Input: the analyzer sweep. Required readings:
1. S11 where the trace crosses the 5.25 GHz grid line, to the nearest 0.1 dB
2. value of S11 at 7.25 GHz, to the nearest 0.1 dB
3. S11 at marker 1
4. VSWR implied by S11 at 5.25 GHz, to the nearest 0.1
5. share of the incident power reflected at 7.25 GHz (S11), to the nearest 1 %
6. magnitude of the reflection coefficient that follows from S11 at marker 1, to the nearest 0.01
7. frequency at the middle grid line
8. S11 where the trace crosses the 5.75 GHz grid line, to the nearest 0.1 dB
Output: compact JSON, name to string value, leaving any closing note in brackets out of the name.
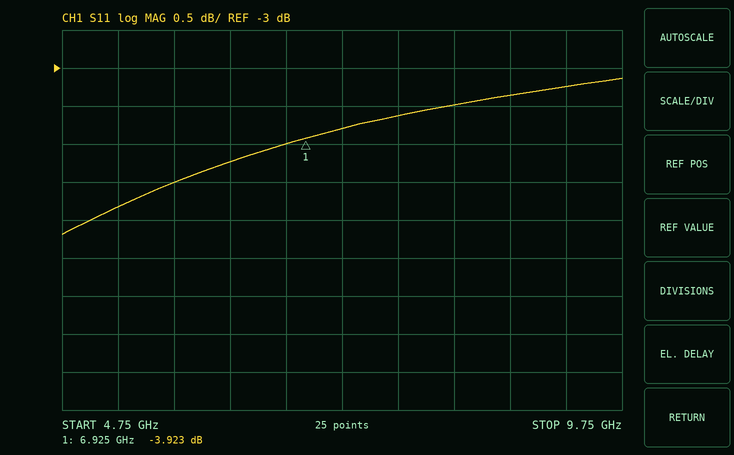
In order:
{"S11 where the trace crosses the 5.25 GHz grid line, to the nearest 0.1 dB": "-4.8 dB", "value of S11 at 7.25 GHz, to the nearest 0.1 dB": "-3.8 dB", "S11 at marker 1": "-3.923 dB", "VSWR implied by S11 at 5.25 GHz, to the nearest 0.1": "3.7", "share of the incident power reflected at 7.25 GHz (S11), to the nearest 1 %": "42 %", "magnitude of the reflection coefficient that follows from S11 at marker 1, to the nearest 0.01": "0.64", "frequency at the middle grid line": "7.25 GHz", "S11 where the trace crosses the 5.75 GHz grid line, to the nearest 0.1 dB": "-4.5 dB"}
